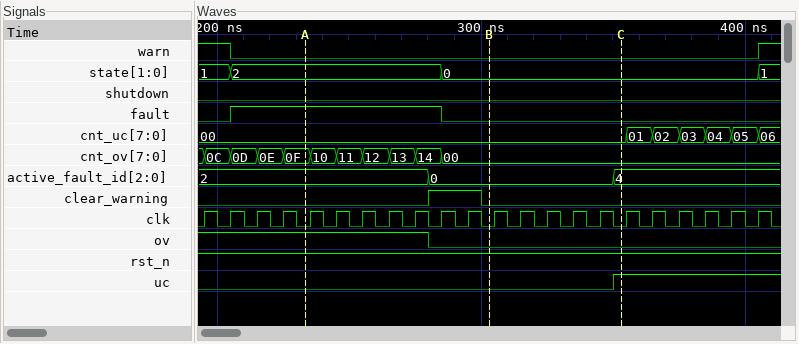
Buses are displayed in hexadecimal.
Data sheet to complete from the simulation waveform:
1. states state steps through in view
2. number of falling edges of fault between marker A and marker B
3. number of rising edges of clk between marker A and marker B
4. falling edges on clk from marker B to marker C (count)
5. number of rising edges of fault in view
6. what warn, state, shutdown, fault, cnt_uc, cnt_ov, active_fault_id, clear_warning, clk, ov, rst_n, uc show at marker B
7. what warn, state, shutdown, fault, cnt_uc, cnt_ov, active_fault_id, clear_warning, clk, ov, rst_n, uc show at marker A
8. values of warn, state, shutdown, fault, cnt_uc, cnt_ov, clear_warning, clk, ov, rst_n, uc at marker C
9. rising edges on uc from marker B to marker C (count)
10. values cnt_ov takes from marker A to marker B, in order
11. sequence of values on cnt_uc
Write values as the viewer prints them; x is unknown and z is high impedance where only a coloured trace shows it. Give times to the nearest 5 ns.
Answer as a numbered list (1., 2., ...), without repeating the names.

1. 1, 2, 0, 1
2. 1
3. 7
4. 5
5. 1
6. warn=0, state=0, shutdown=0, fault=0, cnt_uc=00, cnt_ov=00, active_fault_id=0, clear_warning=0, clk=0, ov=0, rst_n=1, uc=0
7. warn=0, state=2, shutdown=0, fault=1, cnt_uc=00, cnt_ov=0F, active_fault_id=2, clear_warning=0, clk=0, ov=1, rst_n=1, uc=0
8. warn=0, state=0, shutdown=0, fault=0, cnt_uc=00, cnt_ov=00, clear_warning=0, clk=0, ov=0, rst_n=1, uc=1
9. 1
10. 0F, 10, 11, 12, 13, 14, 00
11. 00, 01, 02, 03, 04, 05, 06
